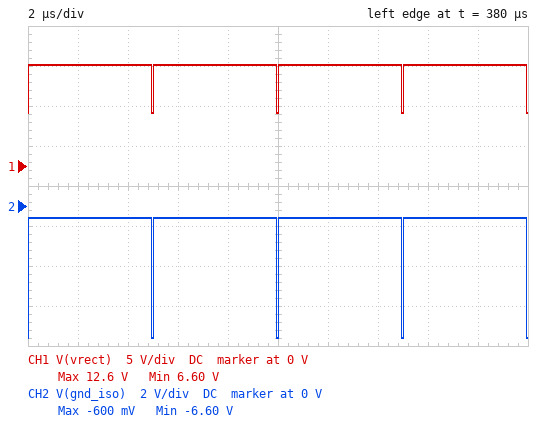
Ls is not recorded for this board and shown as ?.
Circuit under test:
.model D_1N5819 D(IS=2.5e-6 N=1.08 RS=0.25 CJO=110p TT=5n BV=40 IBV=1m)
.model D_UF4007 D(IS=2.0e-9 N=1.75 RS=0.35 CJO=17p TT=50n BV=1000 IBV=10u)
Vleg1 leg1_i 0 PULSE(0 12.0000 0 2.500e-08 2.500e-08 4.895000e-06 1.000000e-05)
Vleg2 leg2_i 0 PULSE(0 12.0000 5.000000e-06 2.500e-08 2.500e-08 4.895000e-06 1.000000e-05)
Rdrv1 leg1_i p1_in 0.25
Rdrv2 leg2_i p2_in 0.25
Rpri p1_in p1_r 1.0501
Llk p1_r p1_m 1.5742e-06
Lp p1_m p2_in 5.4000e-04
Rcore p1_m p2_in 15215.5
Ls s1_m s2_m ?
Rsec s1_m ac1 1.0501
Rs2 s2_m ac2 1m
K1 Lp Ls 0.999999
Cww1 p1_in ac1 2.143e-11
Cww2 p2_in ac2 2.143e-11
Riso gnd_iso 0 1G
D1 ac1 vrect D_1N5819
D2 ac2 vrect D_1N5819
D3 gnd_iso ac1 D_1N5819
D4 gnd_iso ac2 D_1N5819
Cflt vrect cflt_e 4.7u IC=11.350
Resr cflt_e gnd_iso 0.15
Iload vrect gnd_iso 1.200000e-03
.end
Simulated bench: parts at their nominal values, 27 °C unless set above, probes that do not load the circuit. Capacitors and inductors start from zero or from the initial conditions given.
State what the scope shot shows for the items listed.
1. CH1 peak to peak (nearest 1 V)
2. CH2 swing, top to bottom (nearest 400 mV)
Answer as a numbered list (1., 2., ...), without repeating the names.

1. 6 V
2. 6.0 V
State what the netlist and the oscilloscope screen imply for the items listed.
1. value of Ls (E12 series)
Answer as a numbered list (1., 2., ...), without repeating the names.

1. 680 µH
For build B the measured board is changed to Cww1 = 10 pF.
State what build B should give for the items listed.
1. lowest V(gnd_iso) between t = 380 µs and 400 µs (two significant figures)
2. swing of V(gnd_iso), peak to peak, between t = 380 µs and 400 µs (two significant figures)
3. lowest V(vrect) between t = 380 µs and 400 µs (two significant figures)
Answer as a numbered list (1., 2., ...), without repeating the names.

1. -8.3 V
2. 8.0 V
3. 4.9 V
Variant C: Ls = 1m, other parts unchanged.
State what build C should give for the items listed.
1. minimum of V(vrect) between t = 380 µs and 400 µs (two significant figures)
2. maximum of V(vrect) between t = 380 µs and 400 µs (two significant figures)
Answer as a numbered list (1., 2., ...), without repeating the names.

1. 8.1 V
2. 14 V
